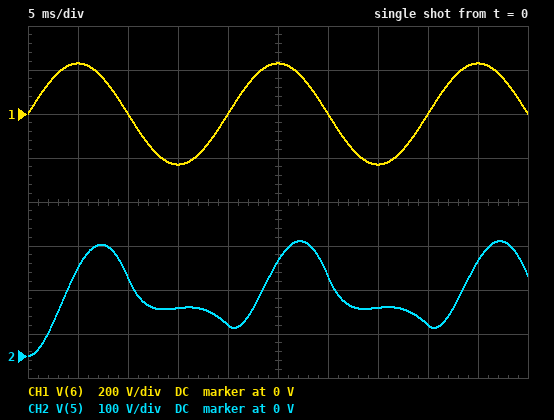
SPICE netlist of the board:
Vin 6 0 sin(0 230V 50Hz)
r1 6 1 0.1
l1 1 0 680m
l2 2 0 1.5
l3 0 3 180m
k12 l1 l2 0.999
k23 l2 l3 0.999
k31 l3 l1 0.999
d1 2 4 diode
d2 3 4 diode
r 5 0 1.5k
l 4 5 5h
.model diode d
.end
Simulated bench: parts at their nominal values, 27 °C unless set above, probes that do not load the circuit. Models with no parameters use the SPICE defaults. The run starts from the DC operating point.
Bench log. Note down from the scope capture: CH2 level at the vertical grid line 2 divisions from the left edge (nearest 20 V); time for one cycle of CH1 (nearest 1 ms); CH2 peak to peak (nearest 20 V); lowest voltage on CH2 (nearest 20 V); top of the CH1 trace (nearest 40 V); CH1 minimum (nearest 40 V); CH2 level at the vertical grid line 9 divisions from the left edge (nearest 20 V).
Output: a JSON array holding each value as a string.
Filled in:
["180 V", "20 ms", "260 V", "0 V", "240 V", "-240 V", "220 V"]
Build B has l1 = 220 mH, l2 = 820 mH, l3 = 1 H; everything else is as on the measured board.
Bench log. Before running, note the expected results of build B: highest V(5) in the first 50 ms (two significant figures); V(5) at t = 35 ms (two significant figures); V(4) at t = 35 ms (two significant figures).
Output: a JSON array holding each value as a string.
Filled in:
["390 V", "340 V", "490 V"]
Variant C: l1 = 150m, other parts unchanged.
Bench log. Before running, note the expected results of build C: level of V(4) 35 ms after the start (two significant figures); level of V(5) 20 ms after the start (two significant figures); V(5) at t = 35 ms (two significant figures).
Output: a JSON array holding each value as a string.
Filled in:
["250 V", "150 V", "230 V"]
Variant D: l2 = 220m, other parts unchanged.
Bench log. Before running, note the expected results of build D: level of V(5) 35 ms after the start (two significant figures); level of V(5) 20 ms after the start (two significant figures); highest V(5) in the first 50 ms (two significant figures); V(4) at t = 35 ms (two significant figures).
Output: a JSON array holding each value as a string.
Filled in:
["85 V", "65 V", "100 V", "120 V"]
